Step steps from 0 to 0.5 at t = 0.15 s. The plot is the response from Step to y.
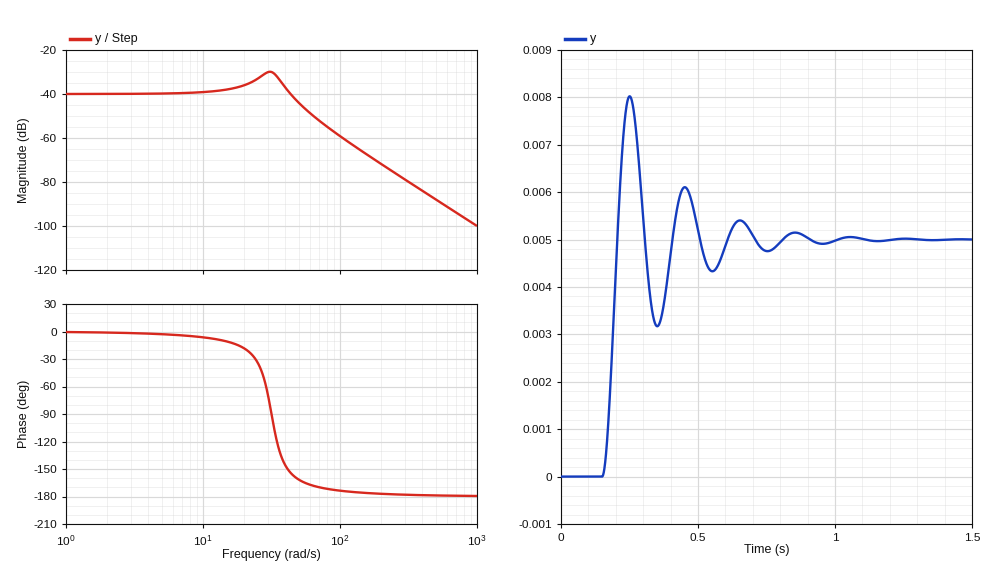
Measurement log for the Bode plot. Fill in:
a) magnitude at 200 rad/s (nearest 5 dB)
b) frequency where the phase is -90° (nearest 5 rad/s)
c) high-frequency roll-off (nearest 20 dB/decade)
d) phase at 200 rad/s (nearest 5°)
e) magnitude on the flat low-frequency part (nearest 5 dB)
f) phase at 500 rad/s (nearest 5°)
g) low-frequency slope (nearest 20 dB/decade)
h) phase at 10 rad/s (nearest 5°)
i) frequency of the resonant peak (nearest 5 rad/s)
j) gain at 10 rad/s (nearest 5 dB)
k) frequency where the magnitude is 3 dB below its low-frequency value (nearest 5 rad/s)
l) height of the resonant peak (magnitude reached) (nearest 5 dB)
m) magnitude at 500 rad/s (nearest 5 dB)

-70 dB
30 rad/s
-40 dB/decade
-175°
-40 dB
-180°
0 dB/decade
-5°
30 rad/s
-40 dB
50 rad/s
-30 dB
-90 dB
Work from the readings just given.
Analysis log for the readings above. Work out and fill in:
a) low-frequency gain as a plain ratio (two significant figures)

0.010
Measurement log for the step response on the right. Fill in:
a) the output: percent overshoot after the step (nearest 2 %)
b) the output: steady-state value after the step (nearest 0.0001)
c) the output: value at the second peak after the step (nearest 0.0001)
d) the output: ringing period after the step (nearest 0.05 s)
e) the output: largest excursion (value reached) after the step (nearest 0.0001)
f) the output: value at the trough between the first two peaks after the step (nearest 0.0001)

60 %
0.0050
0.0061
0.20 s
0.0080
0.0032
